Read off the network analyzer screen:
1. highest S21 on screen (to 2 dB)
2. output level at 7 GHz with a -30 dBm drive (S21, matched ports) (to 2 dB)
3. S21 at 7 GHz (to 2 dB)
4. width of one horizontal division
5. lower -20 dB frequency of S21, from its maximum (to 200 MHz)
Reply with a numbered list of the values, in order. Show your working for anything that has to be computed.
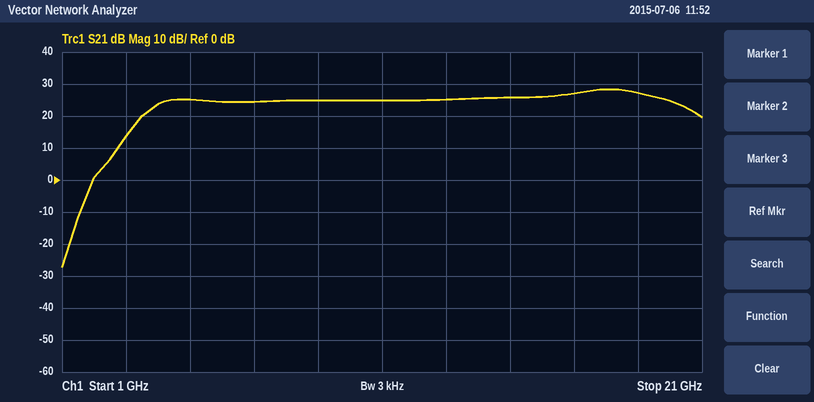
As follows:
1. 28 dB
2. -30 dBm + (24 dB) = -6 dBm
3. 24 dB
4. 2 GHz
5. 2.6 GHz
